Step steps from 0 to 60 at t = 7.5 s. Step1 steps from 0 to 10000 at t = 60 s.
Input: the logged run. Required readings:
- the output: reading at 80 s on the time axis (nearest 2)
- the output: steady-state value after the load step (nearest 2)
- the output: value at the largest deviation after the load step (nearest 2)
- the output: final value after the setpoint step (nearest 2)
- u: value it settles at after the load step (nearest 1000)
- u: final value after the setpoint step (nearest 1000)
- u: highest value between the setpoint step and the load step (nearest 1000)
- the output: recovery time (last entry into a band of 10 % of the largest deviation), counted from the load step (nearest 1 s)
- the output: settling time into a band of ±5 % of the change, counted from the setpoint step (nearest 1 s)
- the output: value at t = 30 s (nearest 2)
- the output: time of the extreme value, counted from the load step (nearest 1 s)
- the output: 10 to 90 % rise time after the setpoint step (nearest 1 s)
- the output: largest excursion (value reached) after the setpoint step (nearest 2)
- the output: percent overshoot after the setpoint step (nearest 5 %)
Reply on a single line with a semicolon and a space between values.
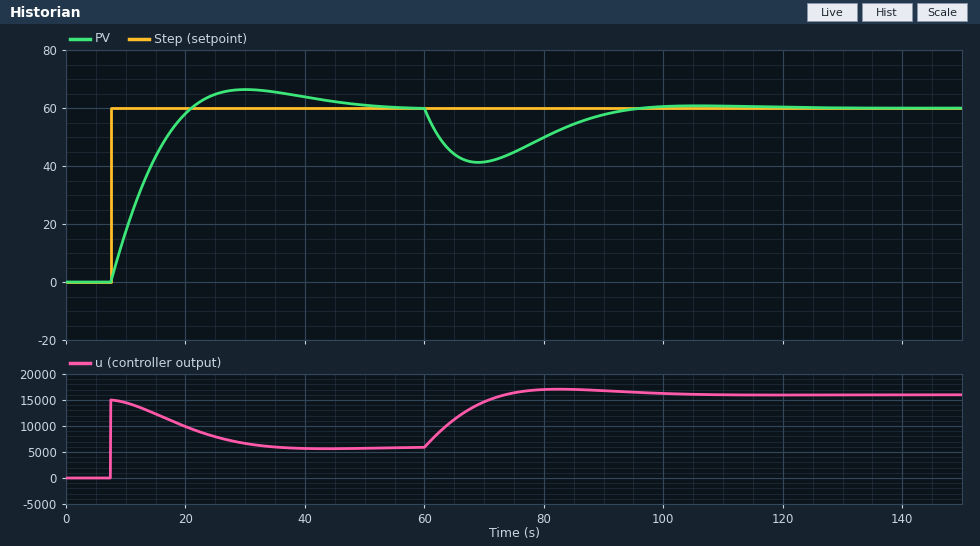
50; 60; 42; 60; 16000; 6000; 15000; 31 s; 35 s; 66; 9 s; 10 s; 66; 10 %
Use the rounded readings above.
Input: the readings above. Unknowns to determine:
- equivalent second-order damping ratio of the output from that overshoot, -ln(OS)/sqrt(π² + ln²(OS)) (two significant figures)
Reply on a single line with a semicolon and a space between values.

0.59
